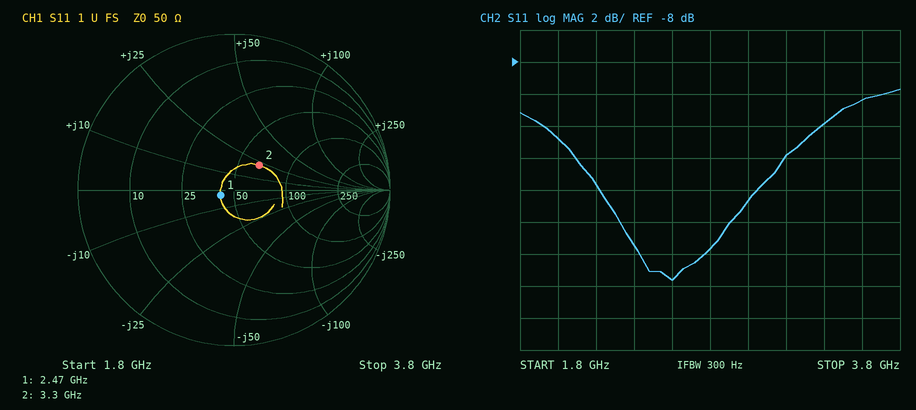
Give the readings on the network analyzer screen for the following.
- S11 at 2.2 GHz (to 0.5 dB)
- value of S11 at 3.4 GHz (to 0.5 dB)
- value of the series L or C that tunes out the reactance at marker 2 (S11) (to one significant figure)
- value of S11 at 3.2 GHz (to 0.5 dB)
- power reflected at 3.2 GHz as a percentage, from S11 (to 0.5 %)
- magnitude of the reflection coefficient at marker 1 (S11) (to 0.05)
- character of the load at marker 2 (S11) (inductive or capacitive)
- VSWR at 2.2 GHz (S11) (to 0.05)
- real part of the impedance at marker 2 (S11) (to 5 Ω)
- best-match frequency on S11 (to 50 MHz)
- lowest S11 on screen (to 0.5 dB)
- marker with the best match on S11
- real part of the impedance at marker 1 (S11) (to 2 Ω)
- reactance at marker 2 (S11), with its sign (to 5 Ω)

-15.5 dB
-12.0 dB
2 pF
-14.0 dB
4.0 %
0.10
inductive
1.40
65 Ω
2.60 GHz
-21.5 dB
marker 1
42 Ω
+20 Ω
